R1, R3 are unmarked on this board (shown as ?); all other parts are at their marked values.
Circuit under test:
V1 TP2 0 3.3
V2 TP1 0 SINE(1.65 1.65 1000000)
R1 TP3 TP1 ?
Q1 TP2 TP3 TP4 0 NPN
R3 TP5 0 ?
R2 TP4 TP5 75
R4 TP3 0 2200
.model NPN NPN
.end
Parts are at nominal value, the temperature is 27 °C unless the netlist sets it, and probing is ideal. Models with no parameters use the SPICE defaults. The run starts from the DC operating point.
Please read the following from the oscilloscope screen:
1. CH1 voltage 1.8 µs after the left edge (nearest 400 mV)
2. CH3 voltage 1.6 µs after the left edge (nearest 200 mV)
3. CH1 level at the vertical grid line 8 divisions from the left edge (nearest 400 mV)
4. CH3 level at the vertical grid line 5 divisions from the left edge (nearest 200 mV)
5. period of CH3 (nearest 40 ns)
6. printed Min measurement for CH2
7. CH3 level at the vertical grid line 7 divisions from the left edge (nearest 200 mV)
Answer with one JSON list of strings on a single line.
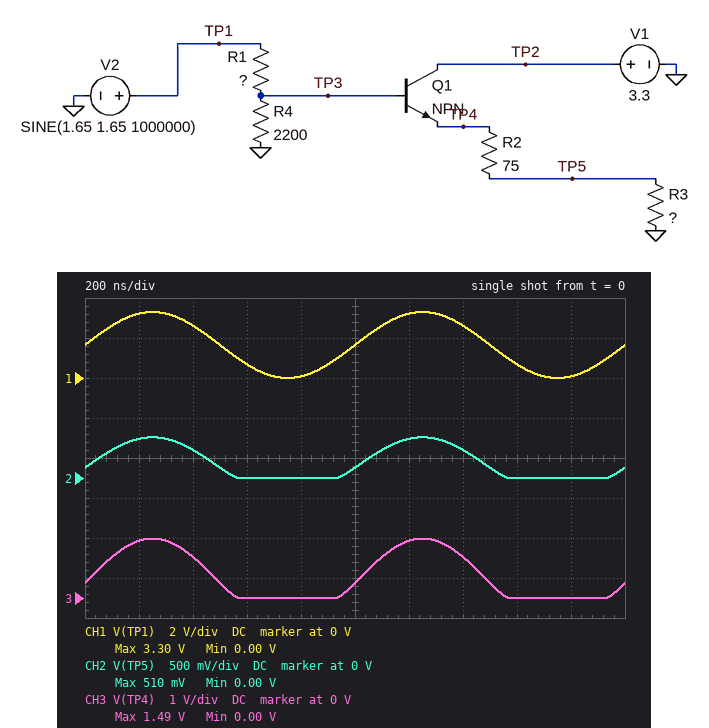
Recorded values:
["0 V", "0 V", "800 mV", "400 mV", "1.00 µs", "0.00 V", "1.0 V"]
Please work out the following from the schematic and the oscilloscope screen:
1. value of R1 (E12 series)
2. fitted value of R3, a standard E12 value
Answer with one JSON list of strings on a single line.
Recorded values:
["820 Ω", "39 Ω"]
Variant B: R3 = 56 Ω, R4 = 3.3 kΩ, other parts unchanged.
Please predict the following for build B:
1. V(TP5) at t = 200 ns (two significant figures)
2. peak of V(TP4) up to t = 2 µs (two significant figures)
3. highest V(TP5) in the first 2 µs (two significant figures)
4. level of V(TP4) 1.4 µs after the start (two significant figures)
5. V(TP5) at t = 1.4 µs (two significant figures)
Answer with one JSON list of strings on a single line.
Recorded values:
["710 mV", "1.7 V", "730 mV", "1.2 V", "520 mV"]
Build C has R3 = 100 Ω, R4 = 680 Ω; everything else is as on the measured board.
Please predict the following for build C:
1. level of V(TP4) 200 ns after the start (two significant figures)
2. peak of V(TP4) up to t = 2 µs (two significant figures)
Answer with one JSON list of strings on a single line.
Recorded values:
["640 mV", "670 mV"]
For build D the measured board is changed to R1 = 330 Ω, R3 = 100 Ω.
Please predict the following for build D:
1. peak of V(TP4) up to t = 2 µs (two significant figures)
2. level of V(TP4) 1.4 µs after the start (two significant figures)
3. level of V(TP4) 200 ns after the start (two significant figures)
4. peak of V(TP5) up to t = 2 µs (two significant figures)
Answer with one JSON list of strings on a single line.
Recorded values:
["2.0 V", "1.4 V", "1.9 V", "1.1 V"]
